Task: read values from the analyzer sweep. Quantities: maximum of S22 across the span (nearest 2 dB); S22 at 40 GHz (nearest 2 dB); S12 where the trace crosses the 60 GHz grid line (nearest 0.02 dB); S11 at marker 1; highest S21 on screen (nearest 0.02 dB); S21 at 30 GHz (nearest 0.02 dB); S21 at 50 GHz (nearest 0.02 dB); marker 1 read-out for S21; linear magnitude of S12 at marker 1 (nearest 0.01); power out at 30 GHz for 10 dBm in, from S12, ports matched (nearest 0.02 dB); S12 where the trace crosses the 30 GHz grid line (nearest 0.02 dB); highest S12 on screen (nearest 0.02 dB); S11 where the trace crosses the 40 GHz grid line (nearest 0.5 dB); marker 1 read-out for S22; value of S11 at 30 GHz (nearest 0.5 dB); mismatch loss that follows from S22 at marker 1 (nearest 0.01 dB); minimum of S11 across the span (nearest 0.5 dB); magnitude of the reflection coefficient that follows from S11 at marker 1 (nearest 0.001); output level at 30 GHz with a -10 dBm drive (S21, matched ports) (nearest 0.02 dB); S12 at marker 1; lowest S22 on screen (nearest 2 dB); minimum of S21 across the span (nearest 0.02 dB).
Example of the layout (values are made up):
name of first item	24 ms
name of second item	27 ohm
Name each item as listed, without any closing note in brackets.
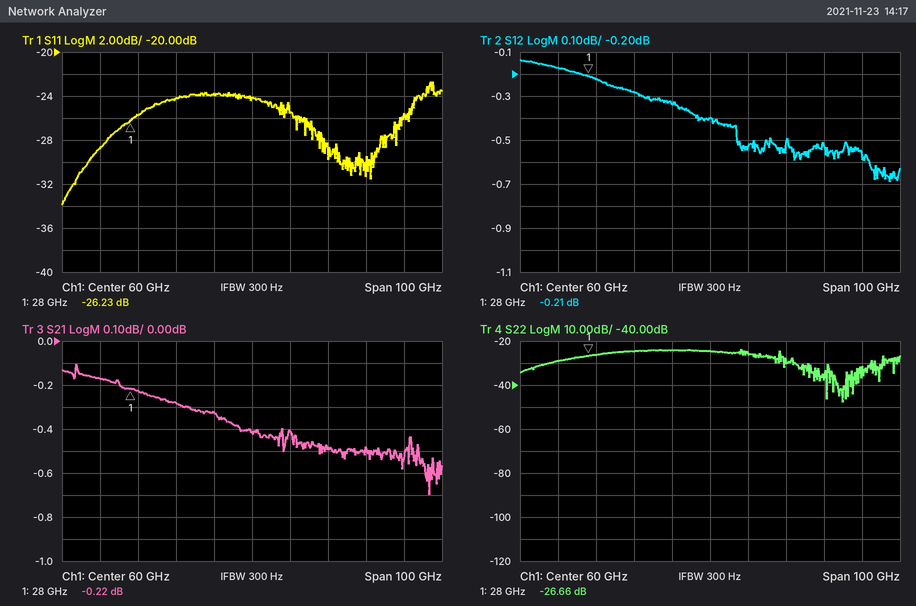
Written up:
maximum of S22 across the span	-24 dB
S22 at 40 GHz	-24 dB
S12 where the trace crosses the 60 GHz grid line	-0.40 dB
S11 at marker 1	-26.23 dB
highest S21 on screen	-0.10 dB
S21 at 30 GHz	-0.22 dB
S21 at 50 GHz	-0.32 dB
marker 1 read-out for S21	-0.22 dB
linear magnitude of S12 at marker 1	0.98
power out at 30 GHz for 10 dBm in, from S12, ports matched	9.78 dBm
S12 where the trace crosses the 30 GHz grid line	-0.22 dB
highest S12 on screen	-0.14 dB
S11 where the trace crosses the 40 GHz grid line	-24.0 dB
marker 1 read-out for S22	-26.66 dB
value of S11 at 30 GHz	-25.5 dB
mismatch loss that follows from S22 at marker 1	0.01 dB
minimum of S11 across the span	-34.0 dB
magnitude of the reflection coefficient that follows from S11 at marker 1	0.049
output level at 30 GHz with a -10 dBm drive (S21, matched ports)	-10.22 dBm
S12 at marker 1	-0.21 dB
lowest S22 on screen	-48 dB
minimum of S21 across the span	-0.70 dB
